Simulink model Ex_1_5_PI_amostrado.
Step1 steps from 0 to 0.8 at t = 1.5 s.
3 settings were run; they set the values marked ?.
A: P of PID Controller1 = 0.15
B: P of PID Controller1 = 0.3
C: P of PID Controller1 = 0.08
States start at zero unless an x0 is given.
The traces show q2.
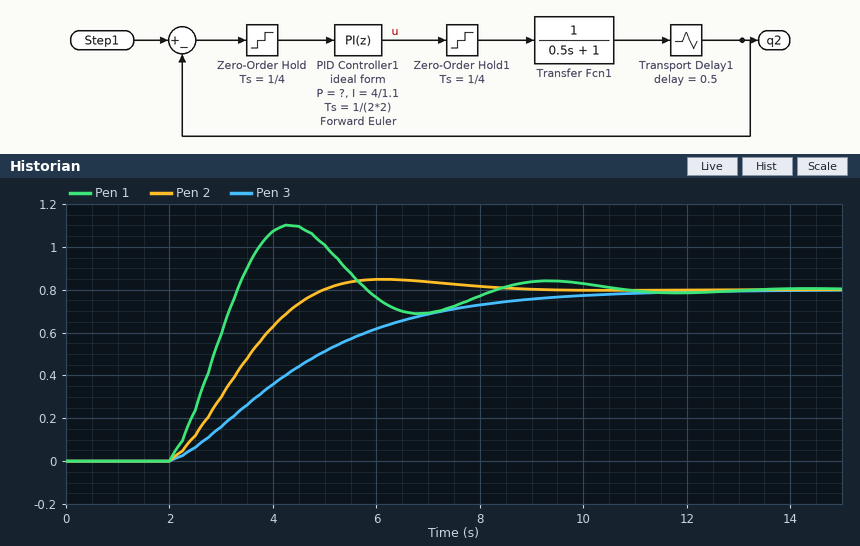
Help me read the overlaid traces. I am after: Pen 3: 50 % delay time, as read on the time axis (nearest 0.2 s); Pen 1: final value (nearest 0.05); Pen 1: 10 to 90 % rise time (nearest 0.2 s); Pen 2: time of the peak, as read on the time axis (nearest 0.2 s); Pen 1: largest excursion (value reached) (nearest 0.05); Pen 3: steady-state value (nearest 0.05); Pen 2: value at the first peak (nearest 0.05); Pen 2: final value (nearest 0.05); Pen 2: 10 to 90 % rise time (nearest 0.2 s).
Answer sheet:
4.2 s
0.80
1.0 s
6.2 s
1.10
0.80
0.85
0.80
2.0 s
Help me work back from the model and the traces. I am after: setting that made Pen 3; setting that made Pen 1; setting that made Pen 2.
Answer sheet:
C
B
A
